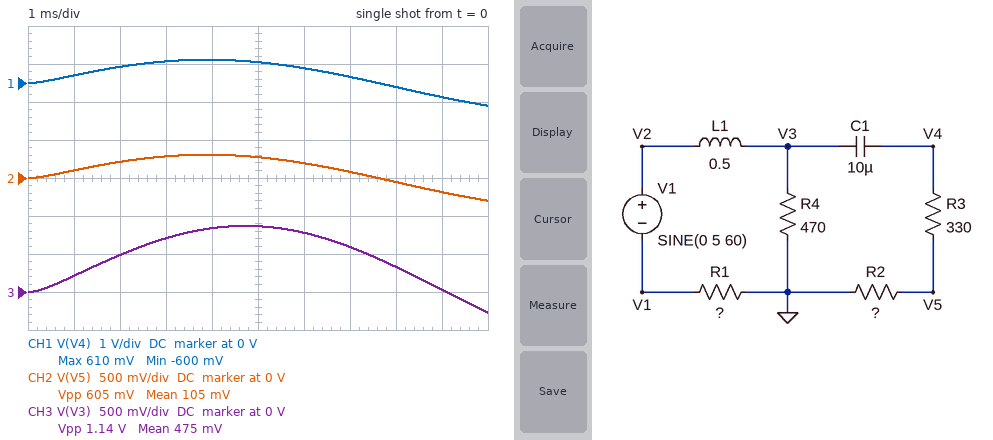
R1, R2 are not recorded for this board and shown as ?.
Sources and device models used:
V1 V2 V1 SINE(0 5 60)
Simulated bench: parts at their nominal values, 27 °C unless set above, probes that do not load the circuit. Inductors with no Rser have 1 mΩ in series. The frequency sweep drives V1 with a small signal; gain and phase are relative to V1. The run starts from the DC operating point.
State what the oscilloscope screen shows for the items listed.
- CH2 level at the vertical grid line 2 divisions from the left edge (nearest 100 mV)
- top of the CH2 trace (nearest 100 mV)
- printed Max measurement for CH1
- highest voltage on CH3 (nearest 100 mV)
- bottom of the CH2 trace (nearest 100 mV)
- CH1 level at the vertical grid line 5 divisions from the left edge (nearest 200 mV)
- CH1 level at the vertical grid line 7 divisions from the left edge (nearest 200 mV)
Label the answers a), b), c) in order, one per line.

a) 200 mV
b) 300 mV
c) 610 mV
d) 900 mV
e) -300 mV
f) 600 mV
g) 200 mV
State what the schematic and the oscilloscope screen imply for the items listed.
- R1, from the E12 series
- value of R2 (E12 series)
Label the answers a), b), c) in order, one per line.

a) 1.5 kΩ
b) 330 Ω
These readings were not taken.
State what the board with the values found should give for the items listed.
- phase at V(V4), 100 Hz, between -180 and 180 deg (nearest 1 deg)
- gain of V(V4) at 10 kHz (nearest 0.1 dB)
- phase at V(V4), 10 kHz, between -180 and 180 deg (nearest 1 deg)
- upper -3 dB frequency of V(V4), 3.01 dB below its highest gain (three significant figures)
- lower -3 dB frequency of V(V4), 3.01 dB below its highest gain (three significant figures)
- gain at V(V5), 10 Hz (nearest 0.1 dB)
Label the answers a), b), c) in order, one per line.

a) -1 deg
b) -41.2 dB
c) -87 deg
d) 594 Hz
e) 14.9 Hz
f) -27.6 dB
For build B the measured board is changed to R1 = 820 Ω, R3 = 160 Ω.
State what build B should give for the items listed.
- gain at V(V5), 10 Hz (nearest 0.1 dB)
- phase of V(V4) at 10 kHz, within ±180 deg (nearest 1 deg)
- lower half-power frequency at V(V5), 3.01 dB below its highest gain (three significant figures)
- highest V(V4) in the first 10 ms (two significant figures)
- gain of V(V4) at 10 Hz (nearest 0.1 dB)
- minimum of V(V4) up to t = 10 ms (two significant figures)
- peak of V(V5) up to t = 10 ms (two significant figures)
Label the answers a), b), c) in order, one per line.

a) -23.4 dB
b) -88 deg
c) 18.3 Hz
d) 840 mV
e) -19.9 dB
f) -850 mV
g) 570 mV
